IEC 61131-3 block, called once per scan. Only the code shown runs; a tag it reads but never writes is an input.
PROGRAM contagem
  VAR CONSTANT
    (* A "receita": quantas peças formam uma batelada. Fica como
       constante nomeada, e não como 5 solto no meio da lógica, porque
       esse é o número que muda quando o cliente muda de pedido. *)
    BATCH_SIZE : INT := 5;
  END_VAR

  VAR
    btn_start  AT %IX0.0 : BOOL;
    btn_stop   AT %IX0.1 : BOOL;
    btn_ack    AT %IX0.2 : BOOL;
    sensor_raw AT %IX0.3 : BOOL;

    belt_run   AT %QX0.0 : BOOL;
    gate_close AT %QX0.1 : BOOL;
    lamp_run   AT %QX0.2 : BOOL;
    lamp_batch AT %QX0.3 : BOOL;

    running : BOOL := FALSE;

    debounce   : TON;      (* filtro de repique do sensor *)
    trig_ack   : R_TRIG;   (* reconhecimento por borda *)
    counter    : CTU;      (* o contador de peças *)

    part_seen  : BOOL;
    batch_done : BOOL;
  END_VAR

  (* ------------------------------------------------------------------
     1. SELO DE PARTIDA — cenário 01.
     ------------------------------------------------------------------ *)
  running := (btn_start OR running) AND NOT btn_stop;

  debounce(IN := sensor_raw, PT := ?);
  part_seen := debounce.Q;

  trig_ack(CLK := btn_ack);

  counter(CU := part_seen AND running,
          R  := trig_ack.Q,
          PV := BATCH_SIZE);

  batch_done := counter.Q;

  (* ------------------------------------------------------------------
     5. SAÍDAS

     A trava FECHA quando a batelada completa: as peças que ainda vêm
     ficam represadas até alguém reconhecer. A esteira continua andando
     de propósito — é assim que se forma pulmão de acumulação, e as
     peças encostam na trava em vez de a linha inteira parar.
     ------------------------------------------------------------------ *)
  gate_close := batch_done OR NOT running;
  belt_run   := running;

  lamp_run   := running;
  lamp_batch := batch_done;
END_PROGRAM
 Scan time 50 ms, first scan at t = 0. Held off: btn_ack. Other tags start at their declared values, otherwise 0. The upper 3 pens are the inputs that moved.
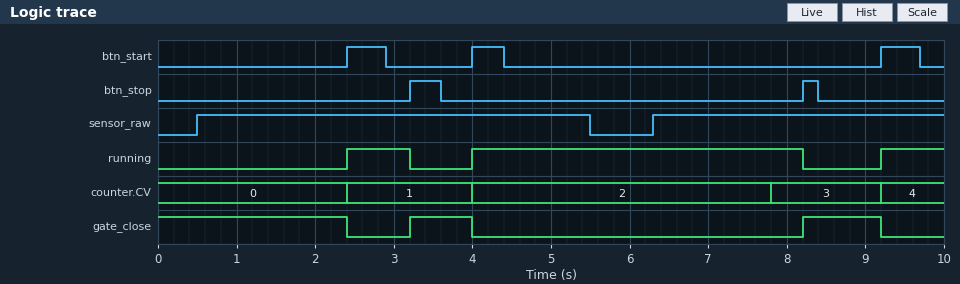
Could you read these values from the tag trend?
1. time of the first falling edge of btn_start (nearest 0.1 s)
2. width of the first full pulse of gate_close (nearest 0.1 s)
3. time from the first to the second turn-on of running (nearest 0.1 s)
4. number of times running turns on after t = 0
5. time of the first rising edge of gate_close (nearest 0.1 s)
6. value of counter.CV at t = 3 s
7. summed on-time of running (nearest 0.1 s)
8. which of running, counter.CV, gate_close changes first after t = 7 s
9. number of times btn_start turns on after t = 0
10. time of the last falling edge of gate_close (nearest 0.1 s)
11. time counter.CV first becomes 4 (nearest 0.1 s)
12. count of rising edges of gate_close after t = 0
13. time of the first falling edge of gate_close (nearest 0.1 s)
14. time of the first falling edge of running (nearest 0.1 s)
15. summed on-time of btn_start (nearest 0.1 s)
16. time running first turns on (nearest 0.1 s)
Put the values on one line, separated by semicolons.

2.9 s; 0.8 s; 1.6 s; 3; 3.2 s; 1; 5.8 s; counter.CV; 3; 9.2 s; 9.2 s; 2; 2.4 s; 3.2 s; 1.4 s; 2.4 s
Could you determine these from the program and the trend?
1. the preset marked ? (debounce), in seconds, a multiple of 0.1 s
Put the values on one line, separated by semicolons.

1.5 s
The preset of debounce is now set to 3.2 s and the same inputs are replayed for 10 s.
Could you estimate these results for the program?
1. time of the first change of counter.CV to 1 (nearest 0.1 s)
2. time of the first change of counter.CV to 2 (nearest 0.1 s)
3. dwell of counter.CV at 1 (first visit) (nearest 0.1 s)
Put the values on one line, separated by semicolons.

4.0 s; 9.5 s; 5.5 s
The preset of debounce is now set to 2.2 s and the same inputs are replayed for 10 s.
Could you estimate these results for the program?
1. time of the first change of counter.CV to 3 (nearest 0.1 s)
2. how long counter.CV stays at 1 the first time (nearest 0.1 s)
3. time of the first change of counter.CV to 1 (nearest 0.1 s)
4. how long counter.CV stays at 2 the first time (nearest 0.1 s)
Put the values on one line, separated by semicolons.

9.2 s; 1.3 s; 2.7 s; 5.2 s
